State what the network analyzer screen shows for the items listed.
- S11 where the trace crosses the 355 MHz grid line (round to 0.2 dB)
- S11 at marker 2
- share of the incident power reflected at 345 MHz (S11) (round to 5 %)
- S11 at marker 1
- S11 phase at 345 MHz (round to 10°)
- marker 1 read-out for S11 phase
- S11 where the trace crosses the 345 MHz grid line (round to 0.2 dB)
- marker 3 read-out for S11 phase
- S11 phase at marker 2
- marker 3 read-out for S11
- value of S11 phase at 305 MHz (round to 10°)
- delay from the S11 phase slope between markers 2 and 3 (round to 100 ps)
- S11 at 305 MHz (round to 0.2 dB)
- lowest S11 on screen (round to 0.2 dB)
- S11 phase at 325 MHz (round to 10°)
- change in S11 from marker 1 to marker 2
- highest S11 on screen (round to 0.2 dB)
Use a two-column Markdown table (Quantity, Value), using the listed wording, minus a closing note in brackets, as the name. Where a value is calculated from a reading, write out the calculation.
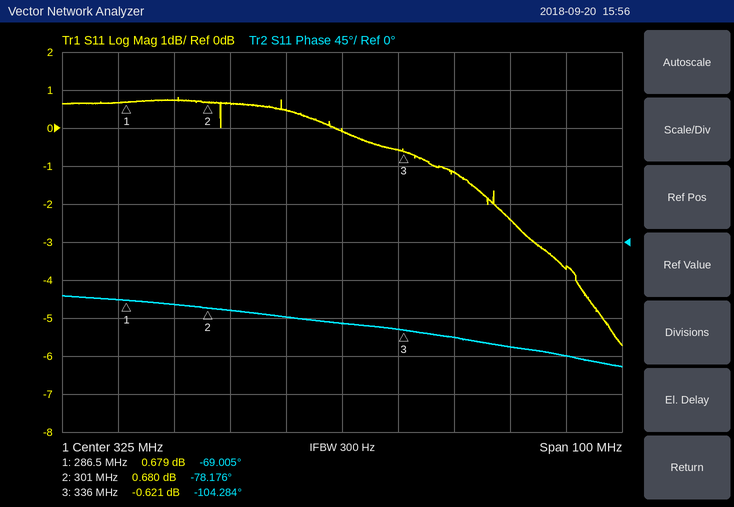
| Quantity | Value |
|---|---|
| S11 where the trace crosses the 355 MHz grid line | -2.4 dB |
| S11 at marker 2 | 0.680 dB |
| share of the incident power reflected at 345 MHz (S11) | 10^(-1.2/10) ≈ 75.9 %, so 75 % to the nearest 5 % |
| S11 at marker 1 | 0.679 dB |
| S11 phase at 345 MHz | -110° |
| marker 1 read-out for S11 phase | -69.005° |
| S11 where the trace crosses the 345 MHz grid line | -1.2 dB |
| marker 3 read-out for S11 phase | -104.284° |
| S11 phase at marker 2 | -78.176° |
| marker 3 read-out for S11 | -0.621 dB |
| value of S11 phase at 305 MHz | -80° |
| delay from the S11 phase slope between markers 2 and 3 | −(-104.284° − (-78.176°))/(360° × 35 MHz) ≈ 2.1 ns |
| S11 at 305 MHz | 0.6 dB |
| lowest S11 on screen | -5.8 dB |
| S11 phase at 325 MHz | -100° |
| change in S11 from marker 1 to marker 2 | 0.68 − (0.679) = 0.001 dB |
| highest S11 on screen | 0.8 dB |
